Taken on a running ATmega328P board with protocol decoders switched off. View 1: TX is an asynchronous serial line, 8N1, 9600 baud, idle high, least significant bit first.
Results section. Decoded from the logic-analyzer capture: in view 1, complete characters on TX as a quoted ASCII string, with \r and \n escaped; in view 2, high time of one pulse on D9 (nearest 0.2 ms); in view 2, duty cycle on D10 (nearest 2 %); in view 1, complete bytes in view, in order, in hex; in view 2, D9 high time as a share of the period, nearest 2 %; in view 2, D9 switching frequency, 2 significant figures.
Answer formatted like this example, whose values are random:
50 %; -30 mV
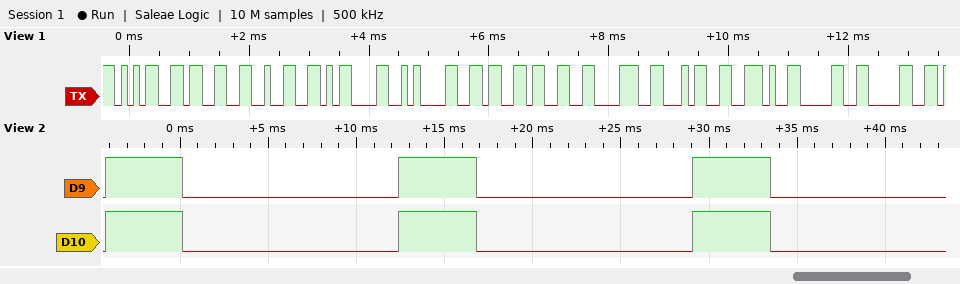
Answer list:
"532\r\n6384.00"; 4.4 ms; 26 %; 35 33 32 0D 0A 36 33 38 34 2E 30 30; 26 %; 60 Hz
